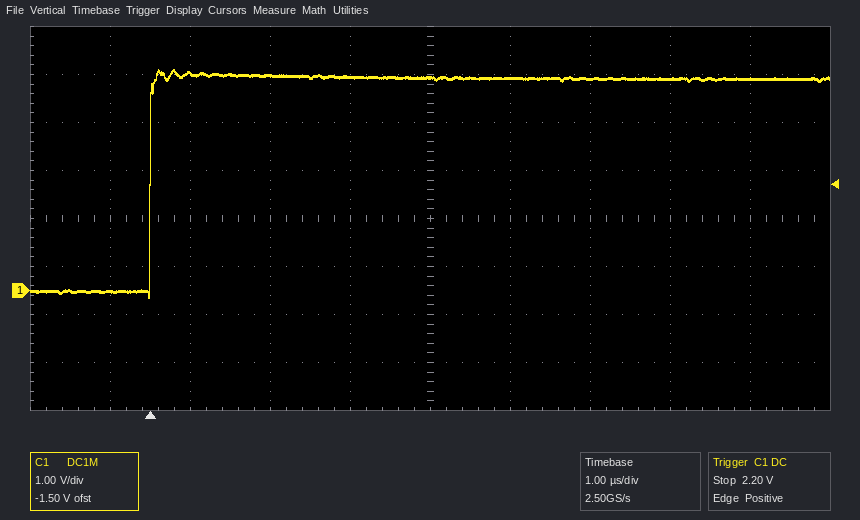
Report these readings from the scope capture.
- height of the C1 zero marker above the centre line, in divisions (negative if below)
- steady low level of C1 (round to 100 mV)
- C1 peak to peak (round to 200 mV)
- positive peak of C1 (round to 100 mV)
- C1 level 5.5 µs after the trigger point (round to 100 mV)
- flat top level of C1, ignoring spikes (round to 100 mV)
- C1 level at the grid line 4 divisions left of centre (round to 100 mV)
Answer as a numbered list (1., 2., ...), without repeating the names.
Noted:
1. -1.5 div
2. 0.0 V
3. 4.8 V
4. 4.6 V
5. 4.4 V
6. 4.4 V
7. 0.0 V
